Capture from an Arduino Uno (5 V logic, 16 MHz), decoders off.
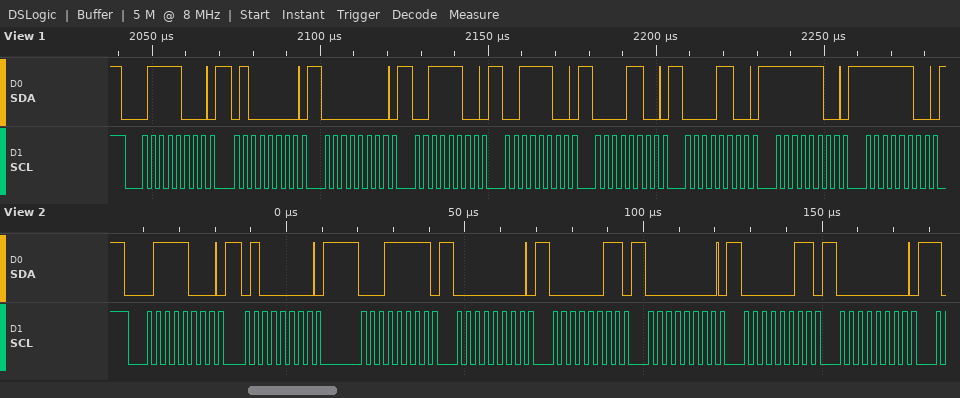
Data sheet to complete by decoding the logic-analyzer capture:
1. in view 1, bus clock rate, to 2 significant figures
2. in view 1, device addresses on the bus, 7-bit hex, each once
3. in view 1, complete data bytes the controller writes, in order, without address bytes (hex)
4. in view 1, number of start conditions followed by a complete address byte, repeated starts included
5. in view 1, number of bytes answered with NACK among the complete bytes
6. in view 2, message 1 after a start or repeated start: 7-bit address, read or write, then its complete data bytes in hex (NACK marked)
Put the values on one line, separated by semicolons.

400 kHz; 0x3C; 40 00 3C 3C 0C 0C FC FC; 1; 0; 0x3C write: 40 1F 00 03 00 03 00
